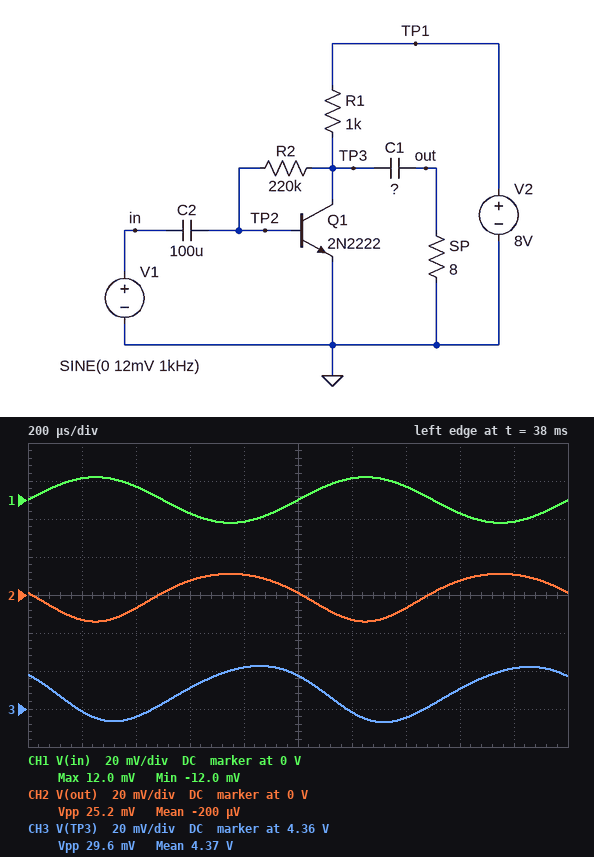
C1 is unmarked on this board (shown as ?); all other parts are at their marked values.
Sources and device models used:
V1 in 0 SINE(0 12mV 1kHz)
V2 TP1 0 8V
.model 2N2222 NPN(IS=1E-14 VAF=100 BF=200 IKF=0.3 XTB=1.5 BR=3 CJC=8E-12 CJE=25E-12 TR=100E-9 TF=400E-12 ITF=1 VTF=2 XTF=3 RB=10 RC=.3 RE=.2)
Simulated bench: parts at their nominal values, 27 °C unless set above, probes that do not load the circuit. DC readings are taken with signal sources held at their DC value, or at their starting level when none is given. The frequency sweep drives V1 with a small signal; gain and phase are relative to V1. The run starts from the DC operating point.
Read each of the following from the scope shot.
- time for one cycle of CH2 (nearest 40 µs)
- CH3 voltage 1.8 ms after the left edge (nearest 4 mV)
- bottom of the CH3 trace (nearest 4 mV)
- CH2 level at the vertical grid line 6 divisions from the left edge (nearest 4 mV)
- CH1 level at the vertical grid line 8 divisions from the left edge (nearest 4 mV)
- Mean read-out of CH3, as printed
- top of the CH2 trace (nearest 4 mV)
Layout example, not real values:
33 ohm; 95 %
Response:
1.00 ms; 4.380 V; 4.352 V; -12 mV; -8 mV; 4.37 V; 12 mV
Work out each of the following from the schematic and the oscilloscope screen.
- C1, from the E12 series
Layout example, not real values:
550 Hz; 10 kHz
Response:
33 µF
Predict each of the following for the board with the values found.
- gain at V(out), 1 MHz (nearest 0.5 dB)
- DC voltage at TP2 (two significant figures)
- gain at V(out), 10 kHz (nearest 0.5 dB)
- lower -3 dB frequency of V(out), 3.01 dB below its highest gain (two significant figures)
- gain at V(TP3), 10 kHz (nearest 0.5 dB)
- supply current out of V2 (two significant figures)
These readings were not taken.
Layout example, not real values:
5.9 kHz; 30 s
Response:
0.5 dB; 690 mV; 0.5 dB; 4.6 Hz; 0.5 dB; 3.5 mA
